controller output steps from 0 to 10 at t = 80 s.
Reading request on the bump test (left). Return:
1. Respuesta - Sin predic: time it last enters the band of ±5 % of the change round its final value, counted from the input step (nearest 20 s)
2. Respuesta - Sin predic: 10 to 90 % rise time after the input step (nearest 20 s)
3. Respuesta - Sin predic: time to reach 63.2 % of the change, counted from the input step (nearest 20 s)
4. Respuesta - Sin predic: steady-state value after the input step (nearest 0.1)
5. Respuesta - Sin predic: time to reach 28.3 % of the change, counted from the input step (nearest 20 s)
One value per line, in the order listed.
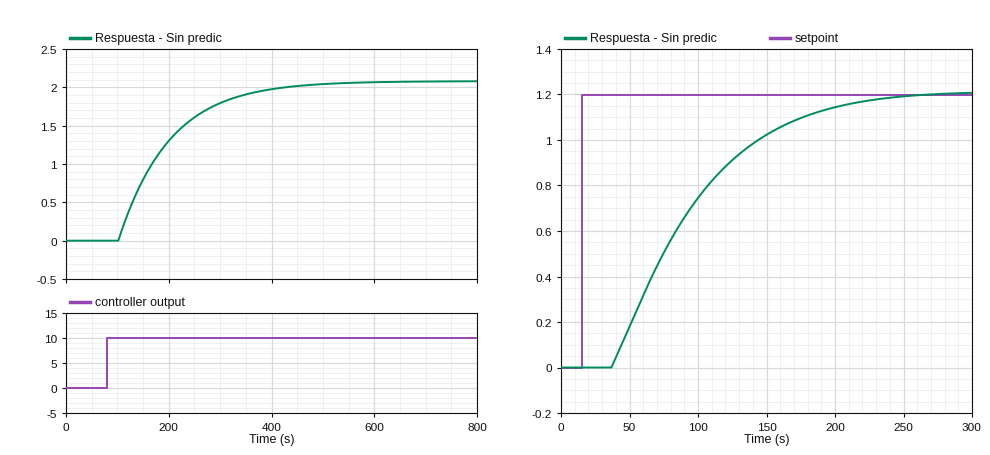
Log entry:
320 s
220 s
120 s
2.1
60 s
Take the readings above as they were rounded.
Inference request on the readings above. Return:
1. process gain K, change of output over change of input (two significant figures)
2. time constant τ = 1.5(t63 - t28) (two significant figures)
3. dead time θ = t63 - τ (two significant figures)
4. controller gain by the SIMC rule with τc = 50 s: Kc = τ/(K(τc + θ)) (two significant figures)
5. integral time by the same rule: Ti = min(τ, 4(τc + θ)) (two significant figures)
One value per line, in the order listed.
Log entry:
0.21
90 s
30 s
5.4
90 s
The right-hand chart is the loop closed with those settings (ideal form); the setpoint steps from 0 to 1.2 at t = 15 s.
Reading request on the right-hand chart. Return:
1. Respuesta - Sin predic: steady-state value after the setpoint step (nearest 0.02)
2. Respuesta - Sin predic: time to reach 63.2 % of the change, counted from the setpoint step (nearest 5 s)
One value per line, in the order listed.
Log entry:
1.20
85 s
